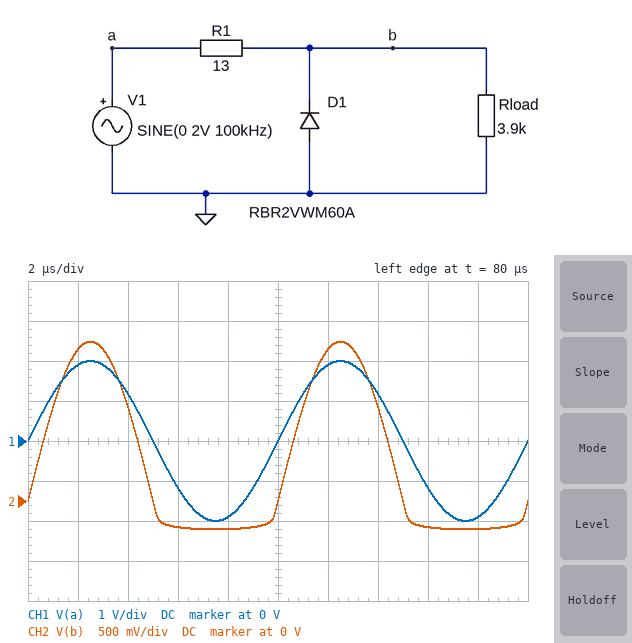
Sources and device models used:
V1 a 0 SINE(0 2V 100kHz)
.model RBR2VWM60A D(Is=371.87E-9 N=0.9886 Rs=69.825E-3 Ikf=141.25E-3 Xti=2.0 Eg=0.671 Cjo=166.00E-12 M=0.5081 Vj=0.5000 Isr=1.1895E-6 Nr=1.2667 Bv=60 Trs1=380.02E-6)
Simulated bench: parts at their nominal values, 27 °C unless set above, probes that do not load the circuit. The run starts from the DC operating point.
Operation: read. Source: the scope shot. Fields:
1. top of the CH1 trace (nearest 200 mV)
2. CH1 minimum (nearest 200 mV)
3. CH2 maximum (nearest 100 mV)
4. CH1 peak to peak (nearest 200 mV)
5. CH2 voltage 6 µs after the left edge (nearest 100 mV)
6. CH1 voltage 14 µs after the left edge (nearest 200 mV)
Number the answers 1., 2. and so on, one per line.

1. 2.0 V
2. -2.0 V
3. 2.0 V
4. 4.0 V
5. -300 mV
6. 1.2 V
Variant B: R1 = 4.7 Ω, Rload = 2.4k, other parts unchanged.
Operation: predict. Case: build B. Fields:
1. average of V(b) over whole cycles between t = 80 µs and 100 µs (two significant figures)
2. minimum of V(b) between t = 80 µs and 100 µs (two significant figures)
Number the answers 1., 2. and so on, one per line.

1. 460 mV
2. -410 mV
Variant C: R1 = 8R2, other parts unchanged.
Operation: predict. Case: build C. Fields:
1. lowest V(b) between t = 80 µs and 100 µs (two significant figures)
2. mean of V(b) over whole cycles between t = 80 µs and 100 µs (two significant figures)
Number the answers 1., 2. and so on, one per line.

1. -380 mV
2. 470 mV
